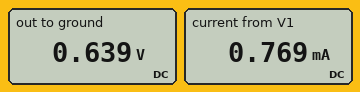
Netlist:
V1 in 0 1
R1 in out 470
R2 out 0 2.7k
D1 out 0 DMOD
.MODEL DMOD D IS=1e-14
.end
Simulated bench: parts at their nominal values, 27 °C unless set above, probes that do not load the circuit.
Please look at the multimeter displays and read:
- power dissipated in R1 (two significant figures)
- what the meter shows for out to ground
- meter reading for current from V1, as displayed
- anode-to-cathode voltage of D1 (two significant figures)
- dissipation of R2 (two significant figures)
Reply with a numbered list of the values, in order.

1. 280 µW
2. 0.639 V
3. 0.769 mA
4. 640 mV
5. 150 µW
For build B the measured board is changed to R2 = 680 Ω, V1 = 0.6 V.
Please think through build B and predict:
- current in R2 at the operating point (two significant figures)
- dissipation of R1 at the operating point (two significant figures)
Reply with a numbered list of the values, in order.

1. 520 µA
2. 130 µW
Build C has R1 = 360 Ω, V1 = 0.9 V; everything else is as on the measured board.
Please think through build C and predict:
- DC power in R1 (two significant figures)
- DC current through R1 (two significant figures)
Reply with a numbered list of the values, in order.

1. 190 µW
2. 730 µA
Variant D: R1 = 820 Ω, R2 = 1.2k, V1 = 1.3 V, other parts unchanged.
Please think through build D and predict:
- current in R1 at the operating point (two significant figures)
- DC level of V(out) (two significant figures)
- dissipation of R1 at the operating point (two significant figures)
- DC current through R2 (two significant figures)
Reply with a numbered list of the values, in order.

1. 820 µA
2. 620 mV
3. 560 µW
4. 520 µA
